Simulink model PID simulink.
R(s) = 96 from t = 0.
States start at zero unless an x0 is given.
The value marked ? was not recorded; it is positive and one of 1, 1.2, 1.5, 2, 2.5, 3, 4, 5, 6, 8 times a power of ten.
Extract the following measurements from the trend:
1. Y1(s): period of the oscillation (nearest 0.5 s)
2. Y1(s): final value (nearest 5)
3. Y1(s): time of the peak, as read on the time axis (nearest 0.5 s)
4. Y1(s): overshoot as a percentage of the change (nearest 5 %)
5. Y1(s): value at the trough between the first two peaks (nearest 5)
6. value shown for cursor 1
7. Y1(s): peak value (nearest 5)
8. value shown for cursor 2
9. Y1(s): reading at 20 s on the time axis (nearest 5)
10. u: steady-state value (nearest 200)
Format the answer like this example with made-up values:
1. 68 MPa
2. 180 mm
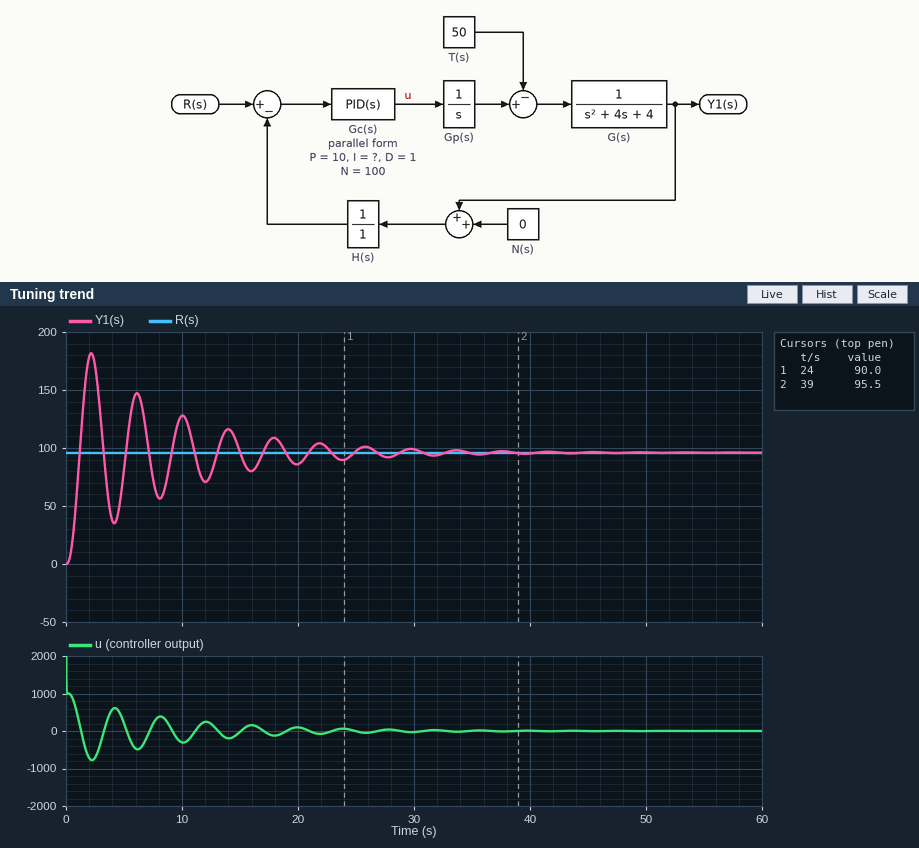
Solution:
1. 4.0 s
2. 95
3. 2.0 s
4. 90 %
5. 35
6. 90.0
7. 180
8. 95.5
9. 85
10. 0
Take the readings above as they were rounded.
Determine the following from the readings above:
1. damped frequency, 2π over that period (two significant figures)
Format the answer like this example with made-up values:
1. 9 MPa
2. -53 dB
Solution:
1. 1.6 rad/s
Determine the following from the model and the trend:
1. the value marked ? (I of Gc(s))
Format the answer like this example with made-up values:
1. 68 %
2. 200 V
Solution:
1. 4
